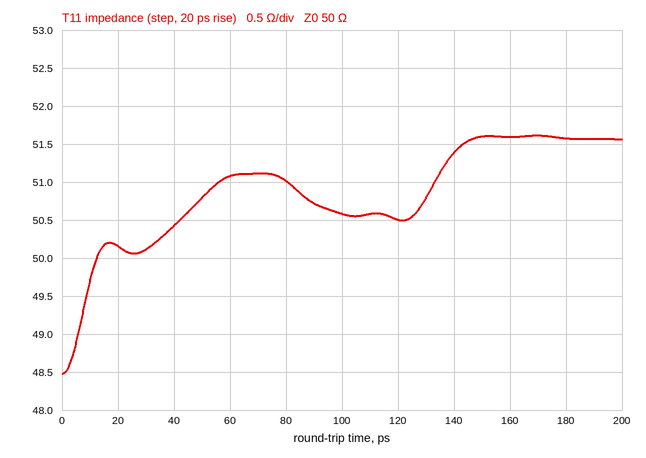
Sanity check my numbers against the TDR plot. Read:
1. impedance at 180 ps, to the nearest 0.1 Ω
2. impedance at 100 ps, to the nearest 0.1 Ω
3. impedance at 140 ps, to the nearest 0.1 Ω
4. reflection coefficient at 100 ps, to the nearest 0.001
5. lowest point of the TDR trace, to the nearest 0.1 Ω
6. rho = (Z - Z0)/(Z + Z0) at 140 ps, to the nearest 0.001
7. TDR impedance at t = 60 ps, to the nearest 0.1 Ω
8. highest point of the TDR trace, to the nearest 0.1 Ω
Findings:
51.6 Ω
50.6 Ω
51.4 Ω
+0.006
48.5 Ω
+0.014
51.1 Ω
51.6 Ω
